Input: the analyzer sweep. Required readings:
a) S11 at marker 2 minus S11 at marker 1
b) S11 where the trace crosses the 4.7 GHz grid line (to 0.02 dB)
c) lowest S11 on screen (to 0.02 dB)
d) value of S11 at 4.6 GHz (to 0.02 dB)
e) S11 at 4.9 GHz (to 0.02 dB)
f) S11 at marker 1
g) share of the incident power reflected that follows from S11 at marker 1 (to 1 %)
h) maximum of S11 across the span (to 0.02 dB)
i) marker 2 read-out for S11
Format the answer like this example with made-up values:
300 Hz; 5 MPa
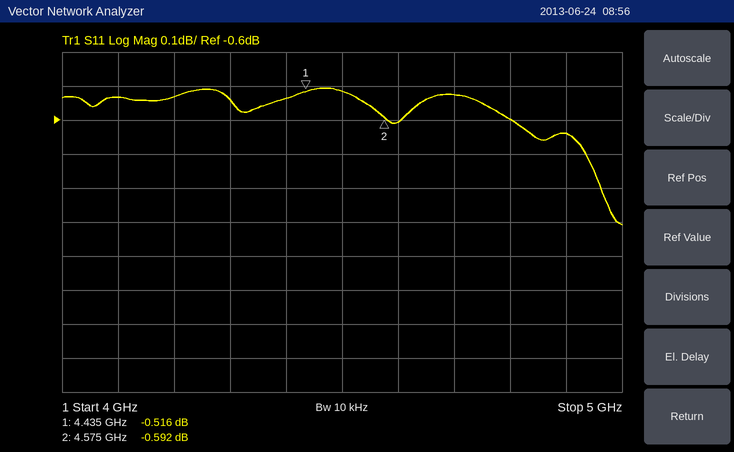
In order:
-0.076 dB; -0.52 dB; -0.90 dB; -0.60 dB; -0.64 dB; -0.516 dB; 89 %; -0.50 dB; -0.592 dB
